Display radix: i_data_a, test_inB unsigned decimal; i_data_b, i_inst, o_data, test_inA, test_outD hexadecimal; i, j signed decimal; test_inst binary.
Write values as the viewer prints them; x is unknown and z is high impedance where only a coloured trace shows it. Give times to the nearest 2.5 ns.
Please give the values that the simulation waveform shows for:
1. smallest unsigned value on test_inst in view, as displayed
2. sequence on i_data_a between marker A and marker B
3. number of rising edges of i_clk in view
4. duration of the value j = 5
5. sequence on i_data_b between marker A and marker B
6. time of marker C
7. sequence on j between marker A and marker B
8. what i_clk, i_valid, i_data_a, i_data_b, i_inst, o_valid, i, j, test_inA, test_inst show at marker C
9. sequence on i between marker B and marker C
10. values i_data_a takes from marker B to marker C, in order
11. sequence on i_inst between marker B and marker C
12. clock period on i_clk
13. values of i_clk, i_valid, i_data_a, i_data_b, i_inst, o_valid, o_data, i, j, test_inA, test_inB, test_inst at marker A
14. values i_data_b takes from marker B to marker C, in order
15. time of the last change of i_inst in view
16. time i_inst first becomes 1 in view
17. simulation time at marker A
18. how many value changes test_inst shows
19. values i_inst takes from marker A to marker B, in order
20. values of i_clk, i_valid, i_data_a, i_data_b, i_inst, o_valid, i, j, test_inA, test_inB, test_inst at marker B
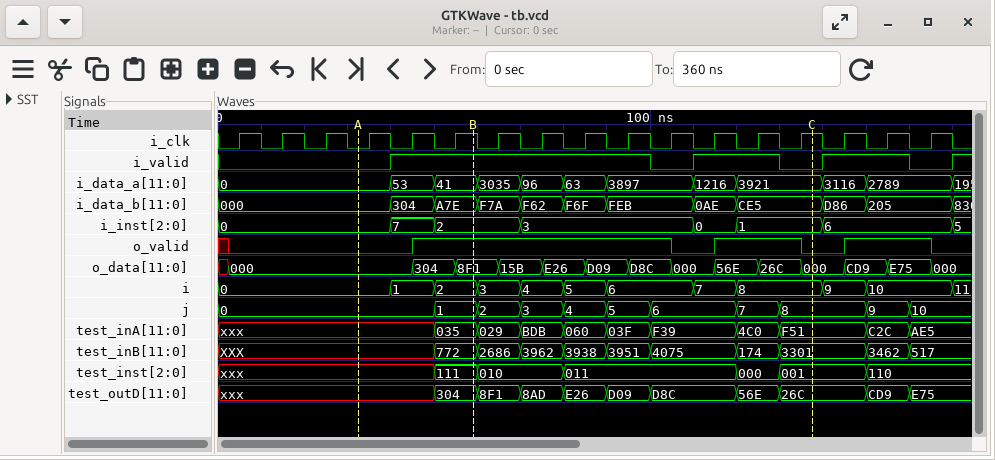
000
0, 53, 41
17
10 ns
000, 304, A7E
137.5 ns
0, 1
i_clk=1, i_valid=0, i_data_a=3921, i_data_b=CE5, i_inst=1, o_valid=0, i=8, j=8, test_inA=F51, test_inst=001
2, 3, 4, 5, 6, 7, 8
41, 3035, 96, 63, 3897, 1216, 3921
2, 3, 0, 1
10 ns
i_clk=0, i_valid=0, i_data_a=0, i_data_b=000, i_inst=0, o_valid=0, o_data=000, i=0, j=0, test_inA=xxx, test_inB=XXX, test_inst=xxx
A7E, F7A, F62, F6F, FEB, 0AE, CE5
170 ns
120 ns
32.5 ns
6
0, 7, 2
i_clk=1, i_valid=1, i_data_a=41, i_data_b=A7E, i_inst=2, o_valid=1, i=2, j=1, test_inA=035, test_inB=772, test_inst=111
